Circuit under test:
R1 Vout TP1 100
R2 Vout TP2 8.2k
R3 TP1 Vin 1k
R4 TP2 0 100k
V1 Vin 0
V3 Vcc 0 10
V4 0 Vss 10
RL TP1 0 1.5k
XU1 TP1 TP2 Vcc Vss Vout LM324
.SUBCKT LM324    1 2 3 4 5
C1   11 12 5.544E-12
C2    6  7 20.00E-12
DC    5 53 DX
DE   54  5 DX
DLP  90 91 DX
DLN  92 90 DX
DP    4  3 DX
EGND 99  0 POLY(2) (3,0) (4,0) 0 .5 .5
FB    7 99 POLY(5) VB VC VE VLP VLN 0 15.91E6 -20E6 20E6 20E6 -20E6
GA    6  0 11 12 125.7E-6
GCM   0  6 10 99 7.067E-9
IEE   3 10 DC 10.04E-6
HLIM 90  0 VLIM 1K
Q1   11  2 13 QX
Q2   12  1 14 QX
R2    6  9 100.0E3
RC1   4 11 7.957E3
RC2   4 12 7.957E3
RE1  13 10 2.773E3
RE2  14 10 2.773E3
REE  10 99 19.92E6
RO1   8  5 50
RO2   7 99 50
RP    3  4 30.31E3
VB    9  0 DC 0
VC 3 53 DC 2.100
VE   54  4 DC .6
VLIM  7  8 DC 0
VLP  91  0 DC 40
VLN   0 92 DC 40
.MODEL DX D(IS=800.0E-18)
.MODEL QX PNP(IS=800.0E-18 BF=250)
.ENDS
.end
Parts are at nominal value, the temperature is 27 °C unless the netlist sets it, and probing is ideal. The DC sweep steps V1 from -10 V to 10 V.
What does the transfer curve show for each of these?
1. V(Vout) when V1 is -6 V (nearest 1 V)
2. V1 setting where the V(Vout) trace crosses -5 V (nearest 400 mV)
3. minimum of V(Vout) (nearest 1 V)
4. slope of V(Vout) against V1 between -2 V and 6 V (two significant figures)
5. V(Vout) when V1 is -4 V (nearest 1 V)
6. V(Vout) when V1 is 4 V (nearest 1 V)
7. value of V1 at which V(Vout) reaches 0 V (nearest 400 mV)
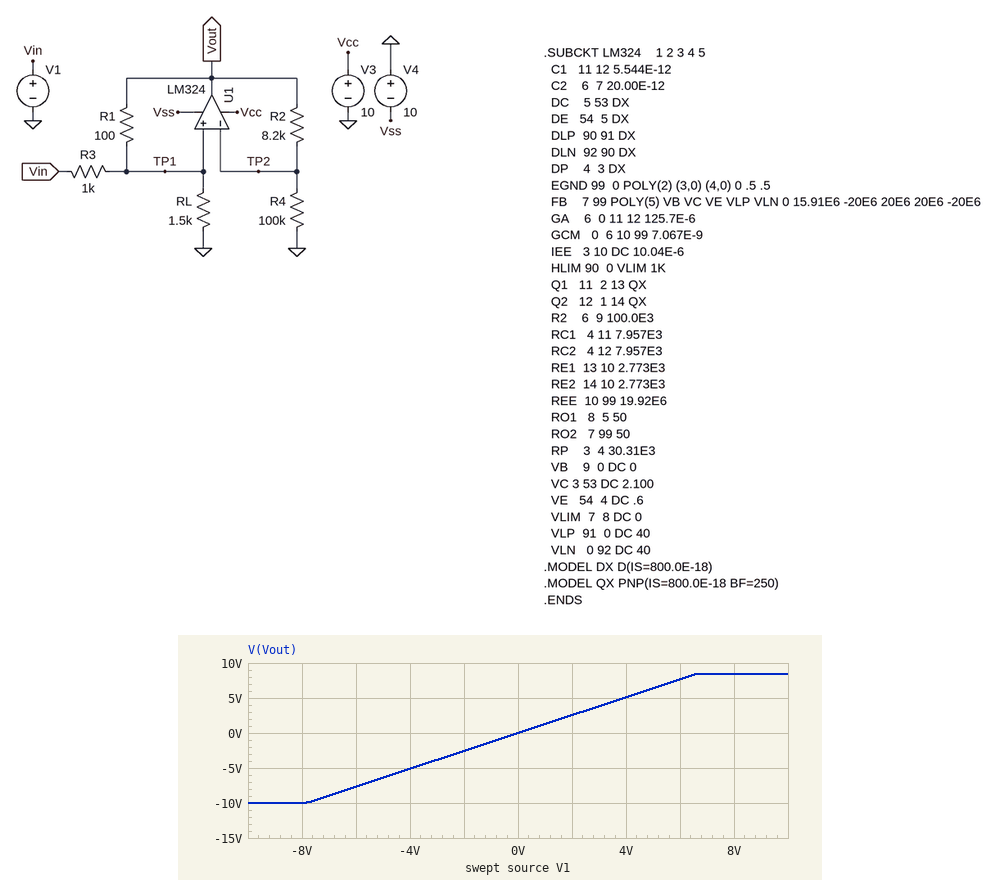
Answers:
-8 V
-4.0 V
-10 V
1.3 V/V
-5 V
5 V
0 V
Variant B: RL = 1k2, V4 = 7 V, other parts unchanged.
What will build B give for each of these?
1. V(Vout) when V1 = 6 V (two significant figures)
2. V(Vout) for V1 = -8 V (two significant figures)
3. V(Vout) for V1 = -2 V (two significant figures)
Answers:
6.4 V
-7.0 V
-2.1 V
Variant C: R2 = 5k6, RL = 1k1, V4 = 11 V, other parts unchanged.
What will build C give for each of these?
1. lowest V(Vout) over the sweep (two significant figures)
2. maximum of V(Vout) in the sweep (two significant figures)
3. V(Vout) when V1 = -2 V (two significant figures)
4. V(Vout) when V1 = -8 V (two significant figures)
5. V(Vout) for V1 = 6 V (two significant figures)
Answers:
-7.8 V
7.8 V
-1.6 V
-6.3 V
4.7 V
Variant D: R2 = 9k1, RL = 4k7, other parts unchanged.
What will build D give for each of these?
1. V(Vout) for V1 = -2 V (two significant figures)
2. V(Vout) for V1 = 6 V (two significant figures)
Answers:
-7.2 V
8.5 V
